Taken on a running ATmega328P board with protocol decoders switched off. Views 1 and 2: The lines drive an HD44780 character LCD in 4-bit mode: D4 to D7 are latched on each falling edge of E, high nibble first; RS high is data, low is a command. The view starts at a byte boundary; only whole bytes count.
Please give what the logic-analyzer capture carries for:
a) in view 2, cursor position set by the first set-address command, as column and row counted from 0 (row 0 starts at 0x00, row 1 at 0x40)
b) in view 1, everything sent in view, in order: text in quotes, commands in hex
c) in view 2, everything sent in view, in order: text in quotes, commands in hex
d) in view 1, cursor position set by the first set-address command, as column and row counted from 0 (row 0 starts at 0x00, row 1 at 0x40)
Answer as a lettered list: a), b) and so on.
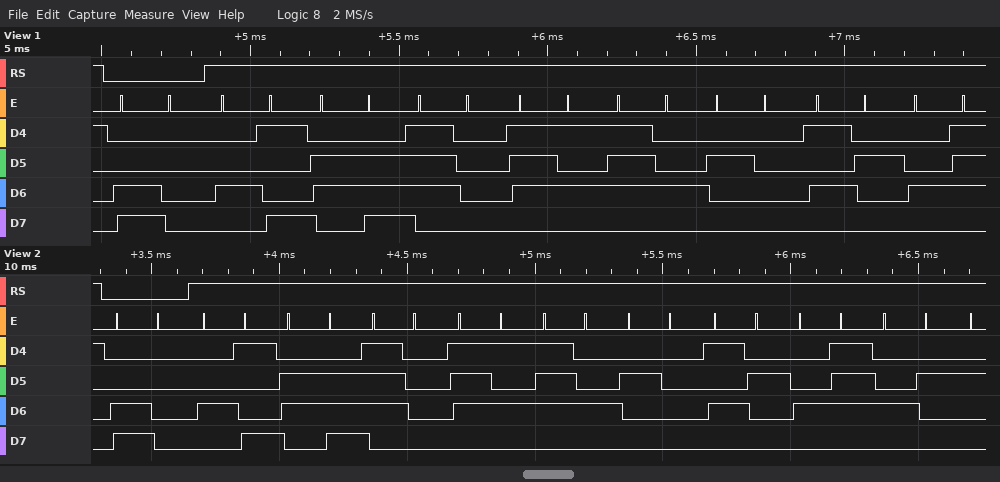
a) column 0, row 1
b) 0xC0 "Input RG"
c) 0xC0 "Input RGB"
d) column 0, row 1
